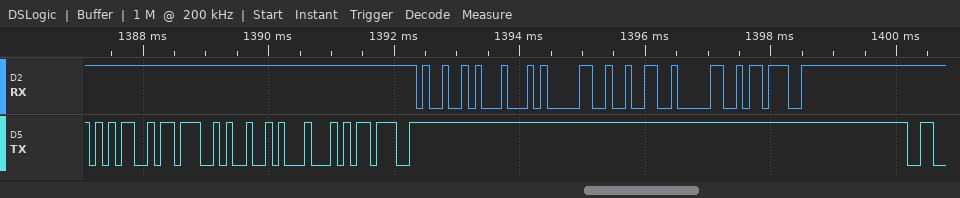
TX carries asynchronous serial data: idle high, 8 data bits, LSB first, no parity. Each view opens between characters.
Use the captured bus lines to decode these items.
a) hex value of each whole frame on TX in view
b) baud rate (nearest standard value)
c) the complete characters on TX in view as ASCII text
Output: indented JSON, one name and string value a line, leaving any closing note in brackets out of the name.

{
  "hex value of each whole frame on TX in view": "35, 3B, 49, 44, 3B",
  "baud rate": "9600 baud",
  "the complete characters on TX in view as ASCII text": "\"5;ID;\""
}
